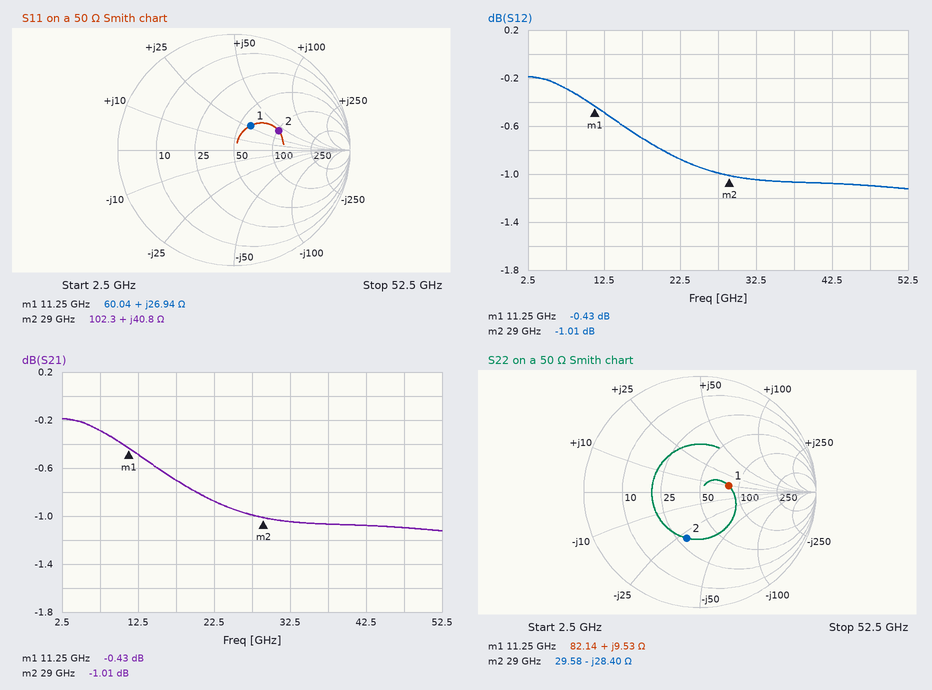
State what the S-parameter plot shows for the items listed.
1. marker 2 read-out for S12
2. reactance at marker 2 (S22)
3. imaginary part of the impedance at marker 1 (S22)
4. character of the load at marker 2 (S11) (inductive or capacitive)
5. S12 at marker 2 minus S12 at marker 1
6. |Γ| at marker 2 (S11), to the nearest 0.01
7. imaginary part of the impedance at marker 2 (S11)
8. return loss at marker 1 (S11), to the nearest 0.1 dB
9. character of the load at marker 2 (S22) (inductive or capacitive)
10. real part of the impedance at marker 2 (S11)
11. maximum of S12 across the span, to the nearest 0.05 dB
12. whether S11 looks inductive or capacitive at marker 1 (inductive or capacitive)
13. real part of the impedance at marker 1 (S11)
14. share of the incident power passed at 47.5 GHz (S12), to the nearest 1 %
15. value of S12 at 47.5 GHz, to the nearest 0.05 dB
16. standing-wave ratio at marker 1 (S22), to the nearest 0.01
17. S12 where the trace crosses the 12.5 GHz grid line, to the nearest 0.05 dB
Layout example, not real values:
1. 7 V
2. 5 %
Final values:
1. -1.01 dB
2. -28.40 Ω
3. +9.53 Ω
4. inductive
5. -0.58 dB
6. 0.42
7. +40.8 Ω
8. 11.9 dB
9. capacitive
10. 102.3 Ω
11. -0.20 dB
12. inductive
13. 60.04 Ω
14. 78 %
15. -1.10 dB
16. 1.68
17. -0.50 dB
